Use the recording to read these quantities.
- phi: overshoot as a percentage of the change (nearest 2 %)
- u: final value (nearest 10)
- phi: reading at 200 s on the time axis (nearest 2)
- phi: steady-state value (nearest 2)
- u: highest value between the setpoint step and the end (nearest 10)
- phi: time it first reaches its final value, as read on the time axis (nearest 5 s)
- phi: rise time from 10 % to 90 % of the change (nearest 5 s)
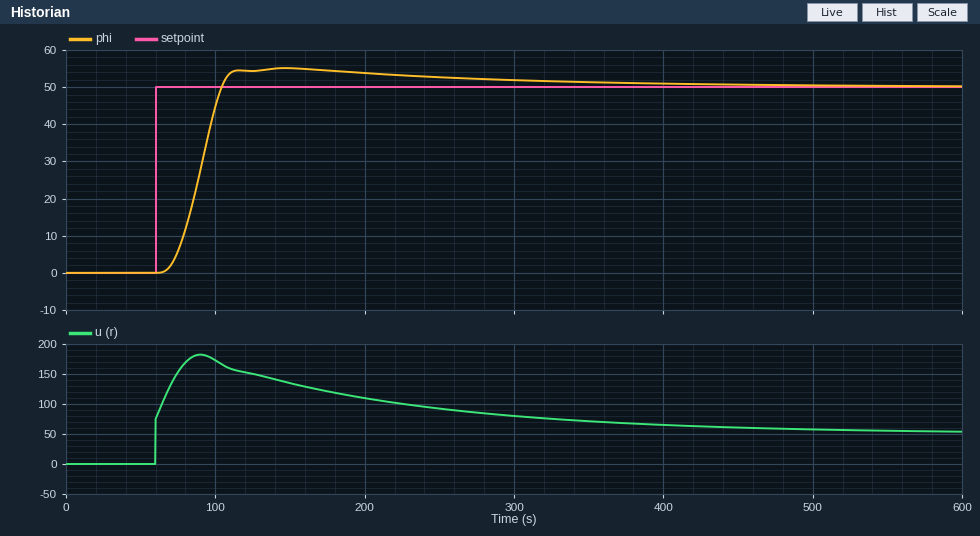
10 %
50
54
50
180
105 s
25 s
